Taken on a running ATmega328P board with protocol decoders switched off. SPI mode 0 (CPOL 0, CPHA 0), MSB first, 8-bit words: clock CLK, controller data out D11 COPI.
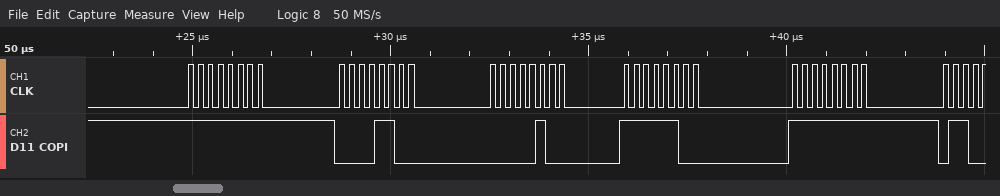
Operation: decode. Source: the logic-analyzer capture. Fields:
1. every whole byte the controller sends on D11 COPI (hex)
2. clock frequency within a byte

0xFF 0x0C 0x04 0xFC 0xFF
4 MHz
